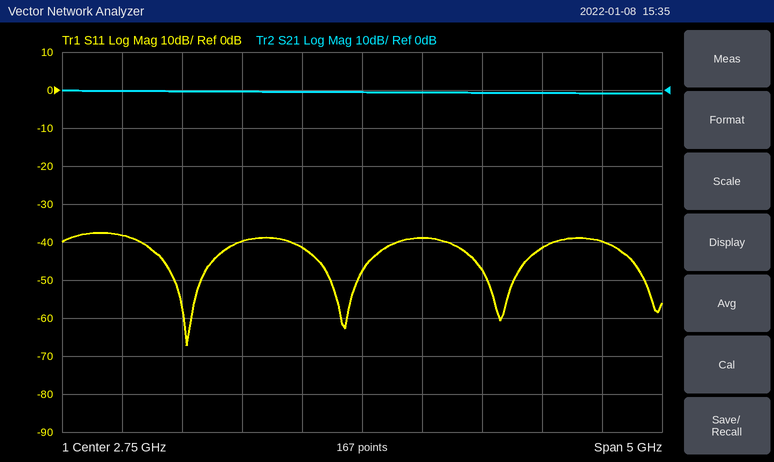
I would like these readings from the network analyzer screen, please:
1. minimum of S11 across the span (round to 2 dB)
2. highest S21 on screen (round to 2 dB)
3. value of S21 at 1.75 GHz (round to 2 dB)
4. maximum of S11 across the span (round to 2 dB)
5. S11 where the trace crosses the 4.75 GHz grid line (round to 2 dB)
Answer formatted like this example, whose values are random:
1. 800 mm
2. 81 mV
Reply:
1. -68 dB
2. 0 dB
3. 0 dB
4. -38 dB
5. -40 dB
